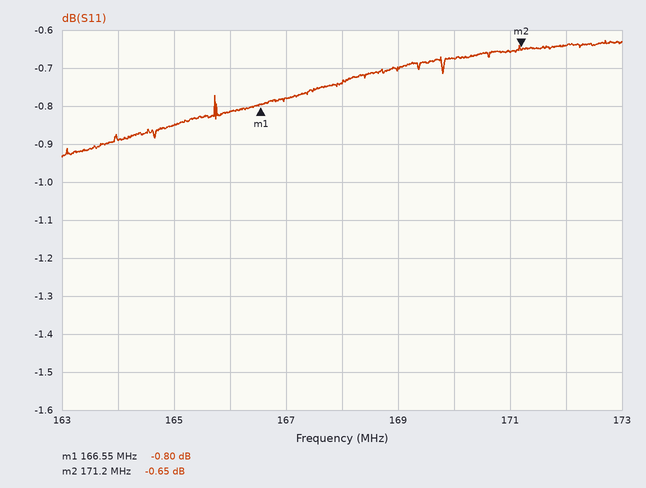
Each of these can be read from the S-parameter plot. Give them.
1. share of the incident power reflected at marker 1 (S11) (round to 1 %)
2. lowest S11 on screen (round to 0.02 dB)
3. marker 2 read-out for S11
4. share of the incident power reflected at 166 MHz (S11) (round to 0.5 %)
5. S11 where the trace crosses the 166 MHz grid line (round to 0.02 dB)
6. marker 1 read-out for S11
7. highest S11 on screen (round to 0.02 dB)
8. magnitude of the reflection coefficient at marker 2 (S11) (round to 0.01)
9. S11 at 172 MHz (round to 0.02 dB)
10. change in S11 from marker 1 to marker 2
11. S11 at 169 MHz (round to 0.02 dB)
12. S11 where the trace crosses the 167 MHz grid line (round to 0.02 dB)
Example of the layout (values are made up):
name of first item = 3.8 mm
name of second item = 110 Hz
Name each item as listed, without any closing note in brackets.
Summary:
share of the incident power reflected at marker 1 (S11) = 83 %
lowest S11 on screen = -0.94 dB
marker 2 read-out for S11 = -0.65 dB
share of the incident power reflected at 166 MHz (S11) = 83.0 %
S11 where the trace crosses the 166 MHz grid line = -0.82 dB
marker 1 read-out for S11 = -0.80 dB
highest S11 on screen = -0.62 dB
magnitude of the reflection coefficient at marker 2 (S11) = 0.93
S11 at 172 MHz = -0.64 dB
change in S11 from marker 1 to marker 2 = 0.15 dB
S11 at 169 MHz = -0.70 dB
S11 where the trace crosses the 167 MHz grid line = -0.78 dB
